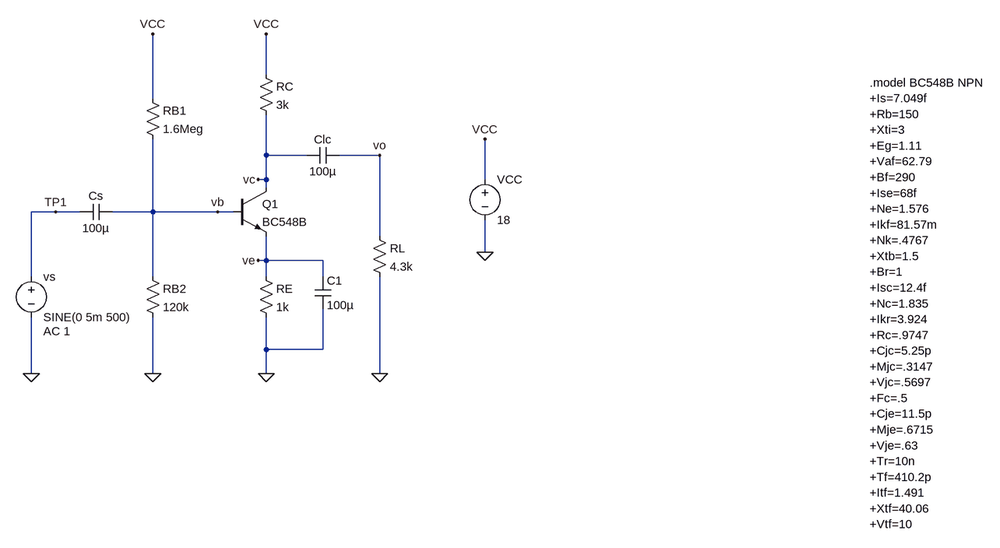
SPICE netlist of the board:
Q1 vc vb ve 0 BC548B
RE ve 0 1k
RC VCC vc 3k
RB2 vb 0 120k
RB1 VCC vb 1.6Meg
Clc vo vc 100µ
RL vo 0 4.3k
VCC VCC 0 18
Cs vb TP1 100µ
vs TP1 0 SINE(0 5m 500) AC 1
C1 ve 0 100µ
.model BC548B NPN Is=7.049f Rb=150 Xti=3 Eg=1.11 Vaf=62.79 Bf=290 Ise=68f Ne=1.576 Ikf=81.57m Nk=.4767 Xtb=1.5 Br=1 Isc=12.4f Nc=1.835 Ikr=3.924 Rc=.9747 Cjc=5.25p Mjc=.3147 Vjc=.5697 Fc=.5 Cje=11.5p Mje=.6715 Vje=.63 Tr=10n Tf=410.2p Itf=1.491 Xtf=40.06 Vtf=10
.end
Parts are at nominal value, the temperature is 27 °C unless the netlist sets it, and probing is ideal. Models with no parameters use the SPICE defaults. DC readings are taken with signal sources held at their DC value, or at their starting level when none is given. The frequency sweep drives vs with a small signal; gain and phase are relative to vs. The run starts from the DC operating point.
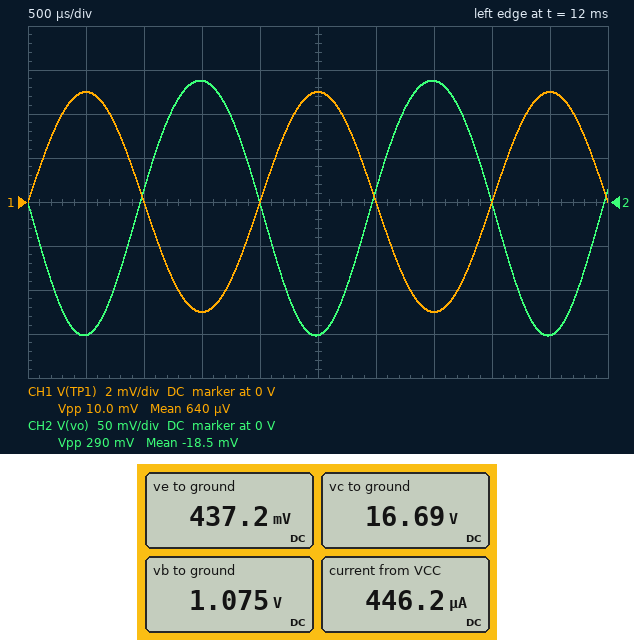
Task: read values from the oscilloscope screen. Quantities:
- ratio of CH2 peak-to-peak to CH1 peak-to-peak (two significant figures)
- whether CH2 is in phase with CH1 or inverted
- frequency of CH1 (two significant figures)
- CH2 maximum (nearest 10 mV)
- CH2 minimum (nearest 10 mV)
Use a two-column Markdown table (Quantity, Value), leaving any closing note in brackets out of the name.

| Quantity | Value |
|---|---|
| ratio of CH2 peak-to-peak to CH1 peak-to-peak | 29 |
| whether CH2 is in phase with CH1 or inverted | inverted |
| frequency of CH1 | 500 Hz |
| CH2 maximum | 140 mV |
| CH2 minimum | -150 mV |
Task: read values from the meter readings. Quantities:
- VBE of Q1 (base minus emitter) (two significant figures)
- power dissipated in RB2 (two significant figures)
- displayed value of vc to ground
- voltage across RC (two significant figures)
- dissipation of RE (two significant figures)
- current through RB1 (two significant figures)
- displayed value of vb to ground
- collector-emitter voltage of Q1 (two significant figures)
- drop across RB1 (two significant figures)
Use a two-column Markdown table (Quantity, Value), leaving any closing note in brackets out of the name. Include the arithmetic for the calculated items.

| Quantity | Value |
|---|---|
| VBE of Q1 (base minus emitter) | 1.075 V - 437.2 mV = 640 mV |
| power dissipated in RB2 | (1.075 V)^2 / 120 kΩ = 9.6 µW |
| displayed value of vc to ground | 16.69 V |
| voltage across RC | 18 V - 16.69 V = 1.3 V |
| dissipation of RE | (437.2 mV)^2 / 1 kΩ = 190 µW |
| current through RB1 | (18 V - 1.075 V) / 1.6 MΩ = 11 µA |
| displayed value of vb to ground | 1.075 V |
| collector-emitter voltage of Q1 | 16.69 V - 437.2 mV = 16 V |
| drop across RB1 | 18 V - 1.075 V = 17 V |
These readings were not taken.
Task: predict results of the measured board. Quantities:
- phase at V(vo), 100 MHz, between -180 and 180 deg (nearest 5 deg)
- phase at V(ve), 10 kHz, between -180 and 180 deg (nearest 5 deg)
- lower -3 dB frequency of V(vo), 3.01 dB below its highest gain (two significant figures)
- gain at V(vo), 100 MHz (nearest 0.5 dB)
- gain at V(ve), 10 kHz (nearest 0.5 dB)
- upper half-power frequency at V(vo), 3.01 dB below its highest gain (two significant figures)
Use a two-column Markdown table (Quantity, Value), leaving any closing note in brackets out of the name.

| Quantity | Value |
|---|---|
| phase at V(vo), 100 MHz, between -180 and 180 deg | 55 deg |
| phase at V(ve), 10 kHz, between -180 and 180 deg | -90 deg |
| lower -3 dB frequency of V(vo), 3.01 dB below its highest gain | 28 Hz |
| gain at V(vo), 100 MHz | 7.5 dB |
| gain at V(ve), 10 kHz | -51.5 dB |
| upper half-power frequency at V(vo), 3.01 dB below its highest gain | 9.9 MHz |
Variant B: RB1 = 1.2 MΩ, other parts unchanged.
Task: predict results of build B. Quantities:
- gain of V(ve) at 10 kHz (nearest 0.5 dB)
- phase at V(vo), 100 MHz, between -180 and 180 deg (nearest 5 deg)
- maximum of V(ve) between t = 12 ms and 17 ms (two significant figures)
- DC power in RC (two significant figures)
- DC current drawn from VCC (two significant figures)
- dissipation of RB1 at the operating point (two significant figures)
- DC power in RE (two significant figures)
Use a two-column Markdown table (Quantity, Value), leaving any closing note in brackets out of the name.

| Quantity | Value |
|---|---|
| gain of V(ve) at 10 kHz | -47.5 dB |
| phase at V(vo), 100 MHz, between -180 and 180 deg | 60 deg |
| maximum of V(ve) between t = 12 ms and 17 ms | 710 mV |
| DC power in RC | 1.5 mW |
| DC current drawn from VCC | 720 µA |
| dissipation of RB1 at the operating point | 230 µW |
| DC power in RE | 500 µW |
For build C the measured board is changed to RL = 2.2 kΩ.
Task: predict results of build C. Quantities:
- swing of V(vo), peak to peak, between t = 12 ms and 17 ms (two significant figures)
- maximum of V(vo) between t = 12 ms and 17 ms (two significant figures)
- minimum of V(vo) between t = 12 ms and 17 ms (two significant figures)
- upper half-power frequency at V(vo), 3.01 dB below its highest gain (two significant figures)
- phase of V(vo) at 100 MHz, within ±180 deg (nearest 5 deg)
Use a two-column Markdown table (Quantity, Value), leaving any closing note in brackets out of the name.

| Quantity | Value |
|---|---|
| swing of V(vo), peak to peak, between t = 12 ms and 17 ms | 210 mV |
| maximum of V(vo) between t = 12 ms and 17 ms | 99 mV |
| minimum of V(vo) between t = 12 ms and 17 ms | -110 mV |
| upper half-power frequency at V(vo), 3.01 dB below its highest gain | 12 MHz |
| phase of V(vo) at 100 MHz, within ±180 deg | 60 deg |
